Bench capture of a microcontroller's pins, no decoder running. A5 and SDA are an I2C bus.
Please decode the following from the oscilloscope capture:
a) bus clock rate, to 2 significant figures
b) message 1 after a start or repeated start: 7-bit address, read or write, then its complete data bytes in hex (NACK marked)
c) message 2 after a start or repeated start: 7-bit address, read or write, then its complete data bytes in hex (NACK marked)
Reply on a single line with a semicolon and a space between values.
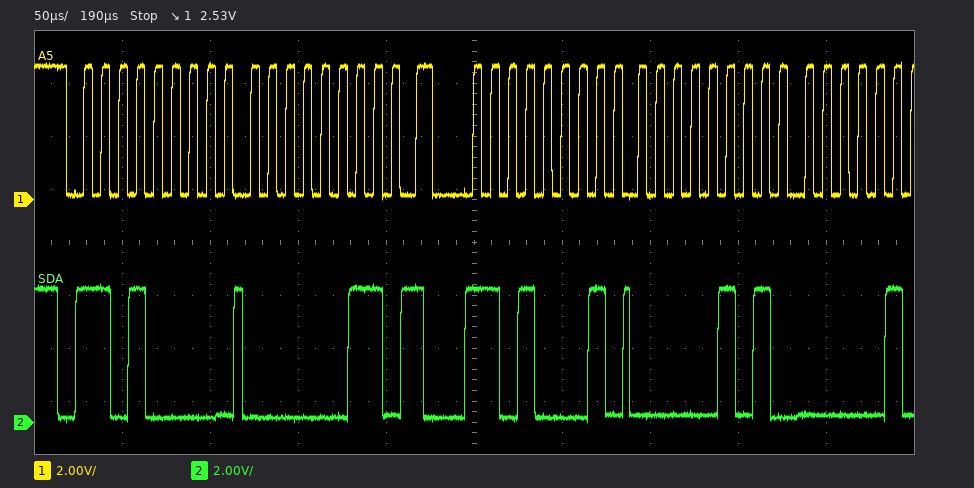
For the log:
100 kHz; 0x68 write: 03; 0x68 read: 05
